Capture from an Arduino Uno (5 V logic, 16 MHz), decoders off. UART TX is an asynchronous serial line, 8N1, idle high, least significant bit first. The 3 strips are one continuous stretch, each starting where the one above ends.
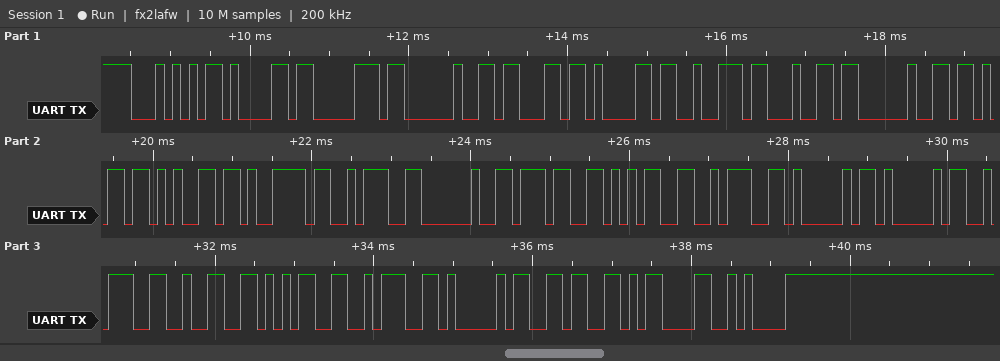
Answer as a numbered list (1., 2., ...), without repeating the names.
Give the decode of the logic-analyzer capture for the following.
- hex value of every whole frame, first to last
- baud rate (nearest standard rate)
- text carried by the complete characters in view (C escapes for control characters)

1. 54 61 70 20 63 61 72 64 20 6B 65 79 3A 20 37 35 3A 41 41 3A 32 35 3A 41 36 0D 0A
2. 9600 baud
3. "Tap card key: 75:AA:25:A6\r\n"
